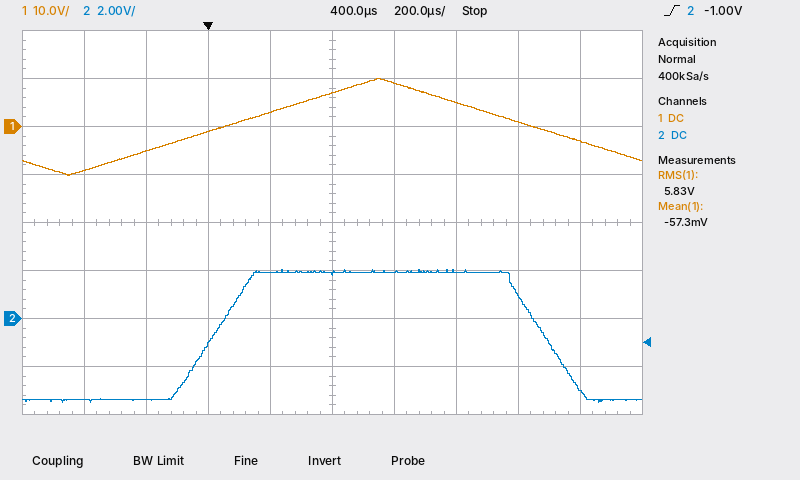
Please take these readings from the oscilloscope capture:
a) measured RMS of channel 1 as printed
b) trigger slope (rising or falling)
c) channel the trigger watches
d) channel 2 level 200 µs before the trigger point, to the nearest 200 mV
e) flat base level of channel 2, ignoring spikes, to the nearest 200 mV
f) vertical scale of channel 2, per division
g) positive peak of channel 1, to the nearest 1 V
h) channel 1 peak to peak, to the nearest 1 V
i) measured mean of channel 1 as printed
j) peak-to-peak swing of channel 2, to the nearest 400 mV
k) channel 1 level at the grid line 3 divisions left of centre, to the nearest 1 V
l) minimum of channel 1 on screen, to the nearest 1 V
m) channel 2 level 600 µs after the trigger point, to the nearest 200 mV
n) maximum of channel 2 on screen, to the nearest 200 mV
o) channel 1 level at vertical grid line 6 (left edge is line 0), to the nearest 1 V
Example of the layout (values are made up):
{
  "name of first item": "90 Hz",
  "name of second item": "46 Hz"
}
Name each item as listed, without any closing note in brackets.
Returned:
{
  "measured RMS of channel 1 as printed": "5.83 V",
  "trigger slope": "rising",
  "channel the trigger watches": "channel 2",
  "channel 2 level 200 µs before the trigger point, to the nearest 200 mV": "-3.4 V",
  "flat base level of channel 2, ignoring spikes, to the nearest 200 mV": "-3.4 V",
  "vertical scale of channel 2, per division": "2 V",
  "positive peak of channel 1, to the nearest 1 V": "10 V",
  "channel 1 peak to peak, to the nearest 1 V": "20 V",
  "measured mean of channel 1 as printed": "-57.3 mV",
  "peak-to-peak swing of channel 2, to the nearest 400 mV": "5.6 V",
  "channel 1 level at the grid line 3 divisions left of centre, to the nearest 1 V": "-5 V",
  "minimum of channel 1 on screen, to the nearest 1 V": "-10 V",
  "channel 2 level 600 µs after the trigger point, to the nearest 200 mV": "2.0 V",
  "maximum of channel 2 on screen, to the nearest 200 mV": "2.0 V",
  "channel 1 level at vertical grid line 6 (left edge is line 0), to the nearest 1 V": "9 V"
}
